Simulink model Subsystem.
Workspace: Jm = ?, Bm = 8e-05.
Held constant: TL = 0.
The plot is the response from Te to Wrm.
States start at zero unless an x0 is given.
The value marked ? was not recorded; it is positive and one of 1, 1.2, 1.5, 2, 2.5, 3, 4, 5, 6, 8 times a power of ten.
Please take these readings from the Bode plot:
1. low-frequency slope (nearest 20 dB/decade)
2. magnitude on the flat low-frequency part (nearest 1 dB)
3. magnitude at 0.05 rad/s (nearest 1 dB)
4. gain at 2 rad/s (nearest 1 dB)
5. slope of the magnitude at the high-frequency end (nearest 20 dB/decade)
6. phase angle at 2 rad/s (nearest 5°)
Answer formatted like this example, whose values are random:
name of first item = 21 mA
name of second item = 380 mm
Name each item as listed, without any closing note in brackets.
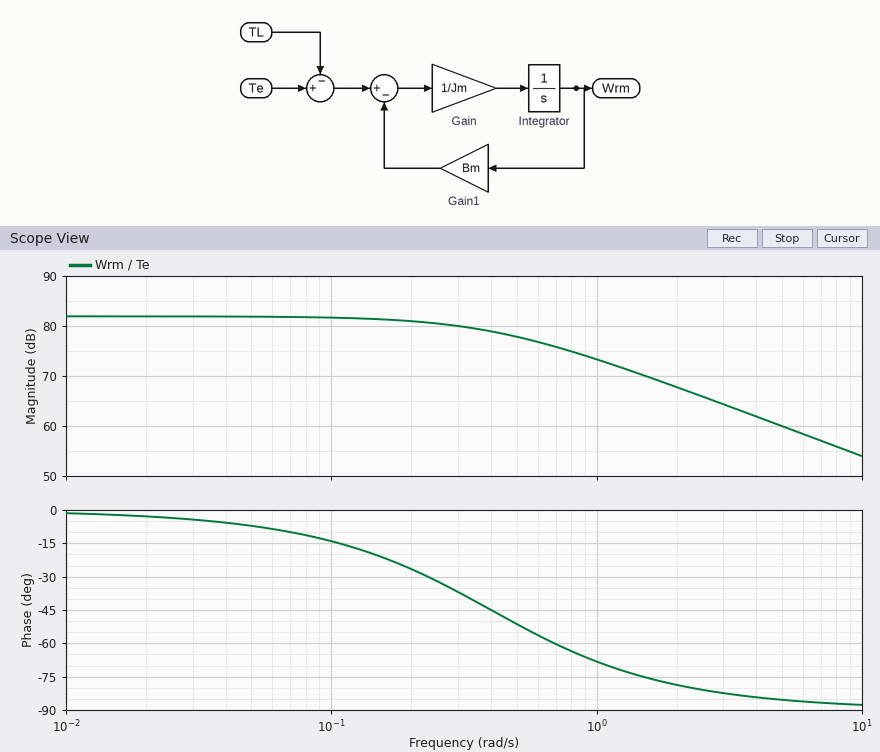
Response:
low-frequency slope = 0 dB/decade
magnitude on the flat low-frequency part = 82 dB
magnitude at 0.05 rad/s = 82 dB
gain at 2 rad/s = 68 dB
slope of the magnitude at the high-frequency end = -20 dB/decade
phase angle at 2 rad/s = -80°
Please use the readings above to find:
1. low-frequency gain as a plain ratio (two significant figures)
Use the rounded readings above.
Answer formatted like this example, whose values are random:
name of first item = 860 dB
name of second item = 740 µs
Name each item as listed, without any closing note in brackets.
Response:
low-frequency gain as a plain ratio = 13000
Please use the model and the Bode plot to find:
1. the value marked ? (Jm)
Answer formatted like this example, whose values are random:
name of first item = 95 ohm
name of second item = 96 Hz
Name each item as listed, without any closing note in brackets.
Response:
the value marked ? = 0.0002
